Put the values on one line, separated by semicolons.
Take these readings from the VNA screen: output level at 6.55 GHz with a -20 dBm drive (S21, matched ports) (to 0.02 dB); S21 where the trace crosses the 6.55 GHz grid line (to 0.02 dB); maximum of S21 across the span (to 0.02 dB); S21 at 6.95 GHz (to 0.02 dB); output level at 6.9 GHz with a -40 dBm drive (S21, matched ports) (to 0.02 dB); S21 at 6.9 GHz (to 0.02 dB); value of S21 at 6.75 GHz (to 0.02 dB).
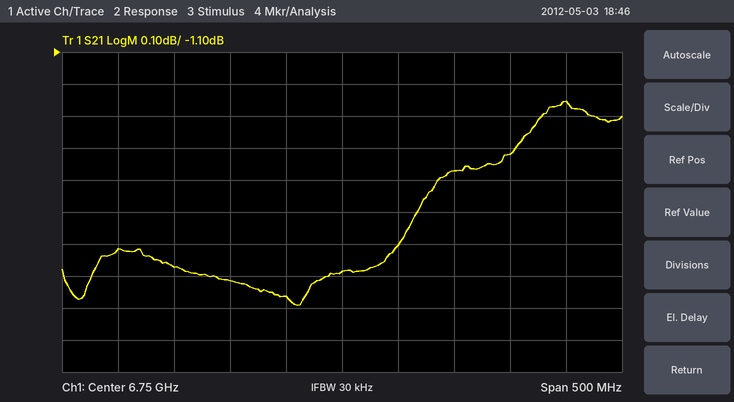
-21.72 dBm; -1.72 dB; -1.26 dB; -1.26 dB; -41.42 dBm; -1.42 dB; -1.78 dB
